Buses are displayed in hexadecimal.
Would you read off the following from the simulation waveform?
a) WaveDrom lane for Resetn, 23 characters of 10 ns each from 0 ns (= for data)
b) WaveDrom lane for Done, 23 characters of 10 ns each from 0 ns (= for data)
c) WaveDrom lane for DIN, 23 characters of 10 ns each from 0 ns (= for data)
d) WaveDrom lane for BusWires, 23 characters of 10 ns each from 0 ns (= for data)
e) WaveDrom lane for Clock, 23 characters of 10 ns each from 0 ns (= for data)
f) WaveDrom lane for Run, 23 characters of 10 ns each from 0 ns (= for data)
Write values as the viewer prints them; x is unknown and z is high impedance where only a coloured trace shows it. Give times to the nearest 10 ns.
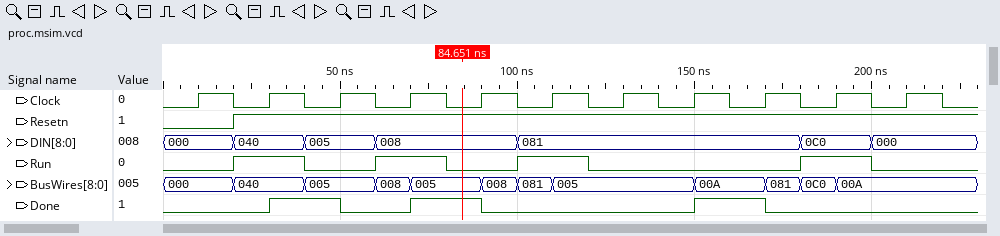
{name: 'Resetn', wave: '0.1....................'}
{name: 'Done', wave: '0..1.0.1.0.....1.0.....'}
{name: 'DIN', wave: '=.=.=.=...=.......=.=..', data: '000 040 005 008 081 0C0 000'}
{name: 'BusWires', wave: '=.=.=.==.===...=.===...', data: '000 040 005 008 005 008 081 005 00A 081 0C0 00A'}
{name: 'Clock', wave: '01010101010101010101010'}
{name: 'Run', wave: '0.1.0.1.0.1.0.....1.0..'}
